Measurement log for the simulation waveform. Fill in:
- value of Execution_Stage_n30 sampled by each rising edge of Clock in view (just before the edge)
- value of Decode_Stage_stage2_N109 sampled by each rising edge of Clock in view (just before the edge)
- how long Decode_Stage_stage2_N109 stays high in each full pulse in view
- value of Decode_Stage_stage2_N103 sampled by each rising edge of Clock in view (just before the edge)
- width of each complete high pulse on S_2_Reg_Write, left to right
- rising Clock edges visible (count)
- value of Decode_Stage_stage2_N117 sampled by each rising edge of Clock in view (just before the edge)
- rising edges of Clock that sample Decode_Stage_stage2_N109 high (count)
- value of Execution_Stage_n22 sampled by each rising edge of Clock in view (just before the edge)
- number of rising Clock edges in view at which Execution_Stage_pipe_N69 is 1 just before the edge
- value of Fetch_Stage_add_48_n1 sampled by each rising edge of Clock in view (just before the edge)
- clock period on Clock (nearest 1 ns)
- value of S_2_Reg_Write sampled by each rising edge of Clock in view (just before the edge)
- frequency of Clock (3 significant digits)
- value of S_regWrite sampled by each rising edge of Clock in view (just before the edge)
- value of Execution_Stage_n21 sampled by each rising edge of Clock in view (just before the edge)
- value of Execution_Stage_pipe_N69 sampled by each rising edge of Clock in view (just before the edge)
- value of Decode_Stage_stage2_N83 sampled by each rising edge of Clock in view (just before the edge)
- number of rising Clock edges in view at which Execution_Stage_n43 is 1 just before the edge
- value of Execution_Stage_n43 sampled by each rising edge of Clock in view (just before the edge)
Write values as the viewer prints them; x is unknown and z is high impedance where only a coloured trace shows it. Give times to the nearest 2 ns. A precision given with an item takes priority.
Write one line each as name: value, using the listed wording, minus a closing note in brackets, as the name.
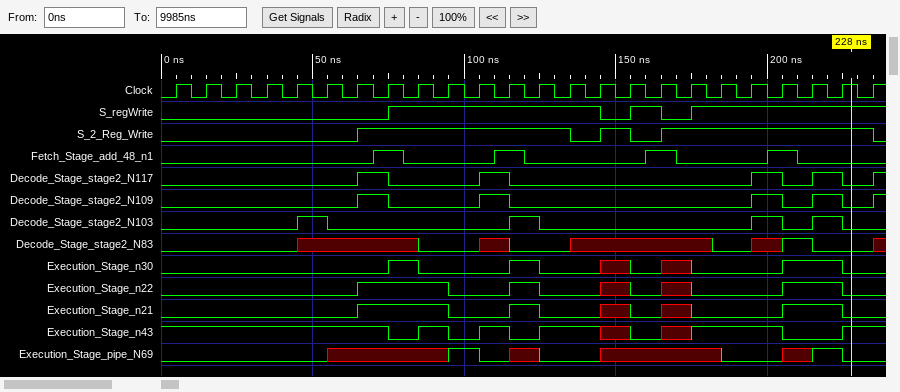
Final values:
value of Execution_Stage_n30 sampled by each rising edge of Clock in view: 0 0 0 0 0 0 0 0 1 0 0 0 1 0 0 x 0 x 0 0 0 1 1 0
value of Decode_Stage_stage2_N109 sampled by each rising edge of Clock in view: 0 0 0 0 0 0 0 1 0 0 0 1 0 0 0 0 0 0 0 0 1 0 1 0
how long Decode_Stage_stage2_N109 stays high in each full pulse in view: 10 ns, 10 ns, 10 ns, 10 ns
value of Decode_Stage_stage2_N103 sampled by each rising edge of Clock in view: 0 0 0 0 0 1 0 0 0 0 0 0 1 0 0 0 0 0 0 0 1 0 1 0
width of each complete high pulse on S_2_Reg_Write, left to right: 70 ns, 10 ns, 70 ns
rising Clock edges visible: 24
value of Decode_Stage_stage2_N117 sampled by each rising edge of Clock in view: 0 0 0 0 0 0 0 1 0 0 0 1 0 0 0 0 0 0 0 0 1 0 1 0
rising edges of Clock that sample Decode_Stage_stage2_N109 high: 4
value of Execution_Stage_n22 sampled by each rising edge of Clock in view: 0 0 0 0 0 0 0 1 1 1 0 0 1 0 0 x 0 x 0 0 0 1 1 0
number of rising Clock edges in view at which Execution_Stage_pipe_N69 is 1 just before the edge: 2
value of Fetch_Stage_add_48_n1 sampled by each rising edge of Clock in view: 0 0 0 0 0 0 0 1 0 0 0 1 0 0 0 0 1 0 0 0 1 0 0 0
clock period on Clock: 10 ns
value of S_2_Reg_Write sampled by each rising edge of Clock in view: 0 0 0 0 0 0 0 1 1 1 1 1 1 1 0 1 0 1 1 1 1 1 1 1
frequency of Clock: 100 MHz
value of S_regWrite sampled by each rising edge of Clock in view: 0 0 0 0 0 0 0 0 1 1 1 1 1 1 1 0 1 0 1 1 1 1 1 1
value of Execution_Stage_n21 sampled by each rising edge of Clock in view: 0 0 0 0 0 0 0 1 1 1 0 0 1 0 0 x 0 x 0 0 0 1 1 0
value of Execution_Stage_pipe_N69 sampled by each rising edge of Clock in view: 0 0 0 0 0 0 x x x x 1 0 x 0 0 x x x x 0 0 x 1 0
value of Decode_Stage_stage2_N83 sampled by each rising edge of Clock in view: 0 0 0 0 0 x x x x 0 0 x 0 0 x x x x 0 0 x 1 0 0
number of rising Clock edges in view at which Execution_Stage_n43 is 1 just before the edge: 16
value of Execution_Stage_n43 sampled by each rising edge of Clock in view: 1 1 1 1 1 1 1 1 0 1 0 1 0 1 1 x 0 x 1 1 1 0 0 1
